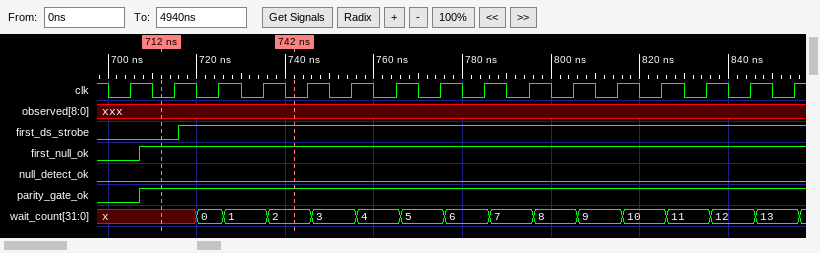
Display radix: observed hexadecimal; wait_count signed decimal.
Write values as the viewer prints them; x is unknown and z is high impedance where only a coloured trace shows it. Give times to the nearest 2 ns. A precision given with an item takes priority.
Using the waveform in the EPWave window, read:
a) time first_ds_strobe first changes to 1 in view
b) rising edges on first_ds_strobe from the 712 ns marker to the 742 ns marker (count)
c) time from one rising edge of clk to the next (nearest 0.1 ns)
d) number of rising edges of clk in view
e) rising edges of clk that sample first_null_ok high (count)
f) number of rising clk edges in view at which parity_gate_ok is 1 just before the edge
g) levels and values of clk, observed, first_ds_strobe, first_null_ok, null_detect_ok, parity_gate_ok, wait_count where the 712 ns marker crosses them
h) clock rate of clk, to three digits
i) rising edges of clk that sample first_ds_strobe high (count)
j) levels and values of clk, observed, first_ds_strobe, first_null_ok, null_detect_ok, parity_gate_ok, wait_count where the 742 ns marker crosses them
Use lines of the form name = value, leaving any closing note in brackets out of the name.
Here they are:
time first_ds_strobe first changes to 1 in view = 716 ns
rising edges on first_ds_strobe from the 712 ns marker to the 742 ns marker = 1
time from one rising edge of clk to the next = 10 ns
number of rising edges of clk in view = 16
rising edges of clk that sample first_null_ok high = 15
number of rising clk edges in view at which parity_gate_ok is 1 just before the edge = 15
levels and values of clk, observed, first_ds_strobe, first_null_ok, null_detect_ok, parity_gate_ok, wait_count where the 712 ns marker crosses them = clk=0, observed=xxx, first_ds_strobe=0, first_null_ok=1, null_detect_ok=0, parity_gate_ok=1, wait_count=x
clock rate of clk, to three digits = 100 MHz
rising edges of clk that sample first_ds_strobe high = 14
levels and values of clk, observed, first_ds_strobe, first_null_ok, null_detect_ok, parity_gate_ok, wait_count where the 742 ns marker crosses them = clk=0, observed=xxx, first_ds_strobe=1, first_null_ok=1, null_detect_ok=0, parity_gate_ok=1, wait_count=2
